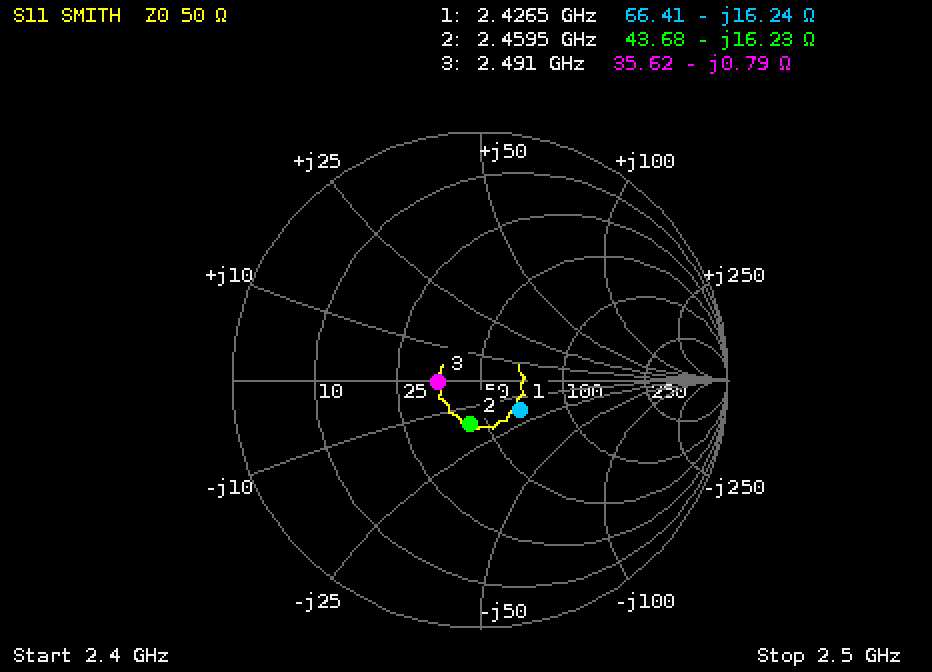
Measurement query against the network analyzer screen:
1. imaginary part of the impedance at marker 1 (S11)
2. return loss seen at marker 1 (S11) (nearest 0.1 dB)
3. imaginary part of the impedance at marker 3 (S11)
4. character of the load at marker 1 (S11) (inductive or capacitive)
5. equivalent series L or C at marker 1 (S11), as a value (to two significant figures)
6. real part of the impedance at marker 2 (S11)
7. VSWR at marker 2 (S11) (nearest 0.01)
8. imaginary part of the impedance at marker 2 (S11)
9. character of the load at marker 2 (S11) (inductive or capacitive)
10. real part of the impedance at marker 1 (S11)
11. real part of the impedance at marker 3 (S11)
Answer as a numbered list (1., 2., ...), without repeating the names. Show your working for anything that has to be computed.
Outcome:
1. -16.24 Ω
2. 14.1 dB
3. -0.79 Ω
4. capacitive
5. C = 1/(2π × 2.4265 GHz × 16.24 Ω) ≈ 4.0 pF
6. 43.68 Ω
7. 1.45
8. -16.23 Ω
9. capacitive
10. 66.41 Ω
11. 35.62 Ω
